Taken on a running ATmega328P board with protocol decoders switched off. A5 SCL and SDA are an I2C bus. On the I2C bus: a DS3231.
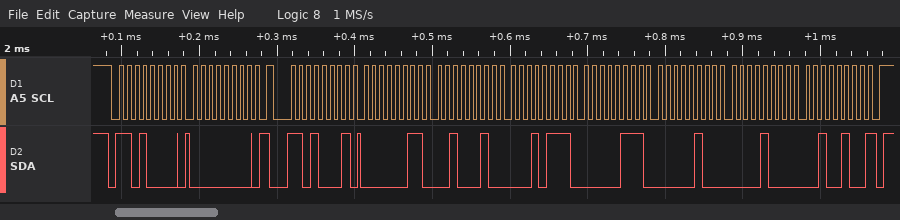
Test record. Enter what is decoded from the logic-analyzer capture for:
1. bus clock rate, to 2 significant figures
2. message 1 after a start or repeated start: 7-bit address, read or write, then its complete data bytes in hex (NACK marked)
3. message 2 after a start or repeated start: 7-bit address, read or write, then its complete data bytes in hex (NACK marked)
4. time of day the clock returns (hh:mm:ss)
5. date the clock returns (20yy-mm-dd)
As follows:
100 kHz
0x68 write: 00
0x68 read: 03 22 17 07 04 08 24 NACK
17:22:03
2024-08-04
